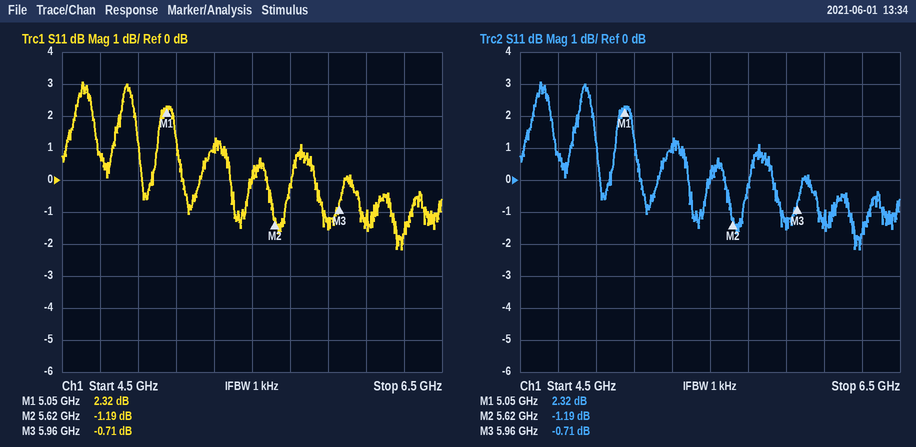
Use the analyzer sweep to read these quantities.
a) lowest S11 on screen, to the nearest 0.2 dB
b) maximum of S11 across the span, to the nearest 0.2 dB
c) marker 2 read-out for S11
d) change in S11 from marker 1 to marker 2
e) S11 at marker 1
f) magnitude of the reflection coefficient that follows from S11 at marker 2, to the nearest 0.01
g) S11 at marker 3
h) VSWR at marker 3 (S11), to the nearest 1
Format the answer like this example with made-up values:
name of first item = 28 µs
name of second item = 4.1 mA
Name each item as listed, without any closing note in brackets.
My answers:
lowest S11 on screen, to the nearest 0.2 dB = -2.2 dB
maximum of S11 across the span, to the nearest 0.2 dB = 3.0 dB
marker 2 read-out for S11 = -1.19 dB
change in S11 from marker 1 to marker 2 = -3.51 dB
S11 at marker 1 = 2.32 dB
magnitude of the reflection coefficient that follows from S11 at marker 2, to the nearest 0.01 = 0.87
S11 at marker 3 = -0.71 dB
VSWR at marker 3 (S11), to the nearest 1 = 24
